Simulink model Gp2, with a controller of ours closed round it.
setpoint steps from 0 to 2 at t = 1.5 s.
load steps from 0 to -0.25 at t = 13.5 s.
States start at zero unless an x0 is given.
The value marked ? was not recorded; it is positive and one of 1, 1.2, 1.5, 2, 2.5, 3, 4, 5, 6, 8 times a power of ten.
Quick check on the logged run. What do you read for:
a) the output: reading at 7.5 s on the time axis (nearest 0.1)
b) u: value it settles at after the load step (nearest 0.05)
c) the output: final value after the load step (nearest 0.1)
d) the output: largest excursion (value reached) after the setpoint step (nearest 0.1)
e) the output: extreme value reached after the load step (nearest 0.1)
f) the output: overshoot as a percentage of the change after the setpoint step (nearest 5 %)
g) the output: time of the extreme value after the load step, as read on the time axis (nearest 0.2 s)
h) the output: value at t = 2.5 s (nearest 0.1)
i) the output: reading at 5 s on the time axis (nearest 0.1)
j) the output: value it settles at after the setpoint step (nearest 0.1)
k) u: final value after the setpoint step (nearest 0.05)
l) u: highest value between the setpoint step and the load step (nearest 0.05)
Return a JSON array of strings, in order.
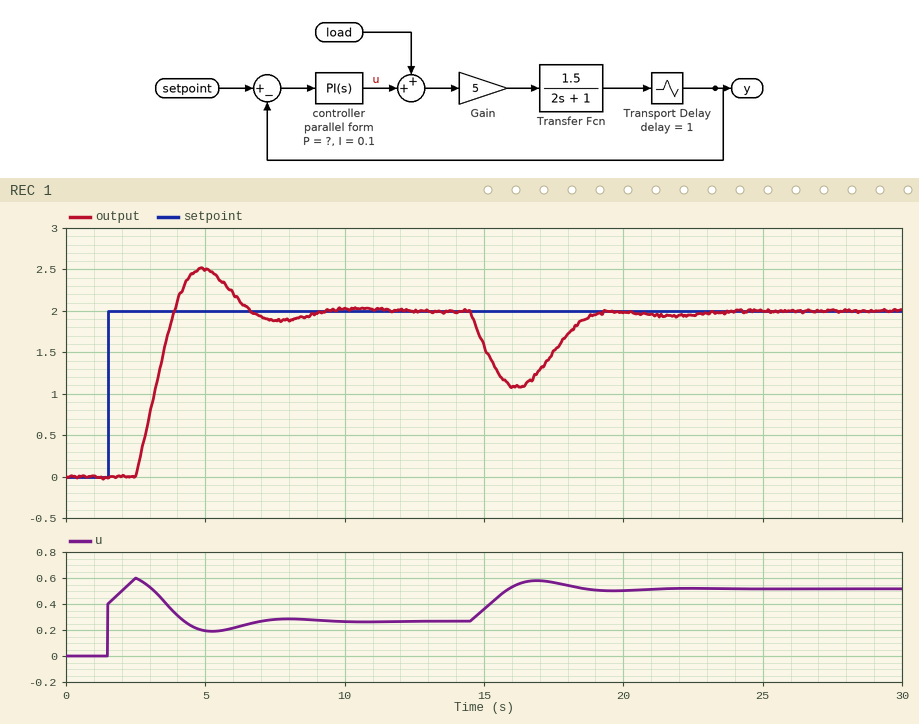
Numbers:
["1.9", "0.50", "2.0", "2.5", "1.1", "25 %", "16.2 s", "0.0", "2.5", "2.0", "0.25", "0.60"]
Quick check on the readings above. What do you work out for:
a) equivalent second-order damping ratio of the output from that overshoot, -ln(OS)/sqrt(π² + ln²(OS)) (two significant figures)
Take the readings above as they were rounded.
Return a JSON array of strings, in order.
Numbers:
["0.40"]
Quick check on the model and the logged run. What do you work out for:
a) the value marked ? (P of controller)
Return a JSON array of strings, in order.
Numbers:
["0.2"]
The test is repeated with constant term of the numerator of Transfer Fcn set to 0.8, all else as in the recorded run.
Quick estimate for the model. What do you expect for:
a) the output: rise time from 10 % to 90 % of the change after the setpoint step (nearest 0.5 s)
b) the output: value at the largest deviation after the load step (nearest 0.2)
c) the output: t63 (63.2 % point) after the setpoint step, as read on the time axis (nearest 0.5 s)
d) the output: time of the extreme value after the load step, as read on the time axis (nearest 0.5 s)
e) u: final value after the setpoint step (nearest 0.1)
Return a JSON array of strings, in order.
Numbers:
["3.0 s", "1.4", "4.0 s", "16.5 s", "0.5"]
